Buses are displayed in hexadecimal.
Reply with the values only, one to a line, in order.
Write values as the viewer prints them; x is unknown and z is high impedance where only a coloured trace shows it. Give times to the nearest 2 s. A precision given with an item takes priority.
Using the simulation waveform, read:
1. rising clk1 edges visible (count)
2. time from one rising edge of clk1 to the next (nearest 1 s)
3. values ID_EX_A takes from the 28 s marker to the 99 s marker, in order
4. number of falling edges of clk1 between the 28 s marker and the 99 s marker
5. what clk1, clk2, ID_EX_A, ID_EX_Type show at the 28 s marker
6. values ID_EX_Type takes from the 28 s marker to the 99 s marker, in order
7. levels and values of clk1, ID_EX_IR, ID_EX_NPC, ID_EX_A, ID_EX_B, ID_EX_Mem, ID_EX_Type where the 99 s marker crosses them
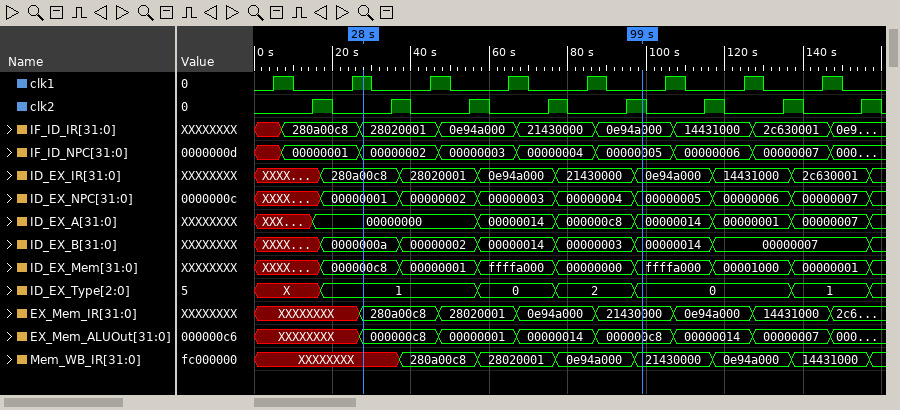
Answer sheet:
8
20 s
00000000, 00000014, 000000c8, 00000014
4
clk1=1, clk2=0, ID_EX_A=00000000, ID_EX_Type=1
1, 0, 2, 0
clk1=0, ID_EX_IR=0e94a000, ID_EX_NPC=00000005, ID_EX_A=00000014, ID_EX_B=00000014, ID_EX_Mem=ffffa000, ID_EX_Type=0
